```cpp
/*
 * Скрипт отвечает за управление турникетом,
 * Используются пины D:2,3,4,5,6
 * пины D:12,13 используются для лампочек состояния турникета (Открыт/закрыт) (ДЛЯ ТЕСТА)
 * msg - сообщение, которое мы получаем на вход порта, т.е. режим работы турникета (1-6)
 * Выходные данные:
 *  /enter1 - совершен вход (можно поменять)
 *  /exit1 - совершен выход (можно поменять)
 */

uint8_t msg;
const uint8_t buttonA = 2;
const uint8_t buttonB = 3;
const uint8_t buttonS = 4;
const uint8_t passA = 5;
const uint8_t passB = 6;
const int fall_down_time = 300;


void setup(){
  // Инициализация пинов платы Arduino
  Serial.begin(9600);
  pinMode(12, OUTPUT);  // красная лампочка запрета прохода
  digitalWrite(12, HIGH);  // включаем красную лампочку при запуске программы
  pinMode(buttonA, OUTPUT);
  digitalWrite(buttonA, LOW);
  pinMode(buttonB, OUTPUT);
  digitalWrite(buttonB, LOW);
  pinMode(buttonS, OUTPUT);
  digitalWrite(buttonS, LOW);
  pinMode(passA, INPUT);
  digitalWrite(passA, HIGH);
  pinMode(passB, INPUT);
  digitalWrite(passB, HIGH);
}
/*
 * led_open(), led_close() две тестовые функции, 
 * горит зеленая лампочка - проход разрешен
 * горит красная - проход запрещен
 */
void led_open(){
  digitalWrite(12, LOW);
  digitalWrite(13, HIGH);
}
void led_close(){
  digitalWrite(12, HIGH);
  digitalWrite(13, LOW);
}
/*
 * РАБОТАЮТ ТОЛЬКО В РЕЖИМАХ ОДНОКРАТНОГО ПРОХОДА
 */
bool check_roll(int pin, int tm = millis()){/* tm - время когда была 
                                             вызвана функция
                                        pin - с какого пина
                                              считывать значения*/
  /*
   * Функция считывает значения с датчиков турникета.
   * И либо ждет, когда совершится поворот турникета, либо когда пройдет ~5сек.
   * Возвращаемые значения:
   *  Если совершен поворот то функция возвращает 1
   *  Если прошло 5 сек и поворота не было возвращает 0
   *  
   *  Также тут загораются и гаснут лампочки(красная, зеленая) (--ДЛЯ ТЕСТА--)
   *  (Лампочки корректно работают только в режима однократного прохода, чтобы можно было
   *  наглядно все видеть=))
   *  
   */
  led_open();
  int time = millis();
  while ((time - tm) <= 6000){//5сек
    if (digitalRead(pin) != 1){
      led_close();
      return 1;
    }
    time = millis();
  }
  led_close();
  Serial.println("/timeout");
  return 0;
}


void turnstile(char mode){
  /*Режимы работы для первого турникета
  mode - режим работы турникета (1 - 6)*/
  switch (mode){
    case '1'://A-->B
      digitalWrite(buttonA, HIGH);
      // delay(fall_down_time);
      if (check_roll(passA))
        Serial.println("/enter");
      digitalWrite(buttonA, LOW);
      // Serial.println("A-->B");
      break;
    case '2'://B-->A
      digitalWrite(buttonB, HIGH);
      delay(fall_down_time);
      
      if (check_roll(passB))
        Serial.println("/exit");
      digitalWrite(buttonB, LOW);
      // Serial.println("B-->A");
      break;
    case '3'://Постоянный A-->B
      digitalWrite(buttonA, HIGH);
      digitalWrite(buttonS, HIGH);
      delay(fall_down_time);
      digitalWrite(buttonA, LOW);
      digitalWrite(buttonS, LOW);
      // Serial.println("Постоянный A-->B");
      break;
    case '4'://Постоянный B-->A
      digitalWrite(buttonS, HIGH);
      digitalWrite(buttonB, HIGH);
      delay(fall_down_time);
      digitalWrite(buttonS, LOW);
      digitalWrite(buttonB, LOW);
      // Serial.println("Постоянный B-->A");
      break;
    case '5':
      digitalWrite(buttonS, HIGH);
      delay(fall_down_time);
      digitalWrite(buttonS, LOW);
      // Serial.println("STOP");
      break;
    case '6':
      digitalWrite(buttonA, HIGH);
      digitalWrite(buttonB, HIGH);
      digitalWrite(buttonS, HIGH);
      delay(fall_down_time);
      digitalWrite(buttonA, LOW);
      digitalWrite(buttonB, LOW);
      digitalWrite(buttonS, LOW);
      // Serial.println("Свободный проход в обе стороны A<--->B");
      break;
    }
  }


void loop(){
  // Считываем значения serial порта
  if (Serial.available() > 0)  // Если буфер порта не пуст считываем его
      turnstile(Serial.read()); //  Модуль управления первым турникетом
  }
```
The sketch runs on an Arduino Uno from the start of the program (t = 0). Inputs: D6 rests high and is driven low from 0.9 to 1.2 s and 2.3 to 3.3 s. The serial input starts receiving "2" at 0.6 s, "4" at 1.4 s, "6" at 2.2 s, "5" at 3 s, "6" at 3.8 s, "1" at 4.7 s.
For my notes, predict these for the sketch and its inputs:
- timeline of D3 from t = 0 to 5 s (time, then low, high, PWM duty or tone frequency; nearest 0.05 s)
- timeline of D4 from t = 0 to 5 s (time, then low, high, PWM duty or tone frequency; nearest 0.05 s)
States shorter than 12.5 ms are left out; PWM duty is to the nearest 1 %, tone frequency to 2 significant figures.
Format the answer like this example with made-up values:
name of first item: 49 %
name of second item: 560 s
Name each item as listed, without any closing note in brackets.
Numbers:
timeline of D3 from t = 0 to 5 s: 0 s low; 0.6 s high; 0.9 s low; 1.4 s high; 1.7 s low; 2.2 s high; 2.5 s low; 3.8 s high; 4.1 s low
timeline of D4 from t = 0 to 5 s: 0 s low; 1.4 s high; 1.7 s low; 2.2 s high; 2.5 s low; 3 s high; 3.3 s low; 3.8 s high; 4.1 s low
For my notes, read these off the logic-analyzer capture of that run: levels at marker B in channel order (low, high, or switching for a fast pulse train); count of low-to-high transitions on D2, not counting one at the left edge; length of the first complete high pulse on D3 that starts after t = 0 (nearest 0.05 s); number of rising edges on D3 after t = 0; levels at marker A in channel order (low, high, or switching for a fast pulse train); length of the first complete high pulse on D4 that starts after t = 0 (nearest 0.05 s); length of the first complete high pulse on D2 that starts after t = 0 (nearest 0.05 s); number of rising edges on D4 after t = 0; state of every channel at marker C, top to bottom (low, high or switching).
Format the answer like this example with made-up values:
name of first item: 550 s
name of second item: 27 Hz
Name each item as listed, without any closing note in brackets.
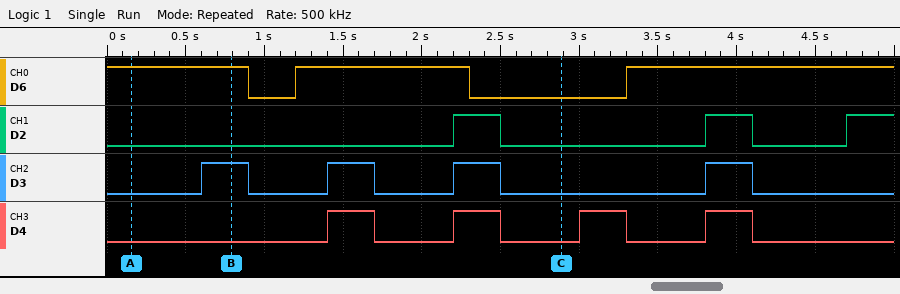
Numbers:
levels at marker B in channel order: D6 high, D2 low, D3 high, D4 low
count of low-to-high transitions on D2, not counting one at the left edge: 3
length of the first complete high pulse on D3 that starts after t = 0: 0.30 s
number of rising edges on D3 after t = 0: 4
levels at marker A in channel order: D6 high, D2 low, D3 low, D4 low
length of the first complete high pulse on D4 that starts after t = 0: 0.30 s
length of the first complete high pulse on D2 that starts after t = 0: 0.30 s
number of rising edges on D4 after t = 0: 4
state of every channel at marker C, top to bottom: D6 low, D2 low, D3 low, D4 low
